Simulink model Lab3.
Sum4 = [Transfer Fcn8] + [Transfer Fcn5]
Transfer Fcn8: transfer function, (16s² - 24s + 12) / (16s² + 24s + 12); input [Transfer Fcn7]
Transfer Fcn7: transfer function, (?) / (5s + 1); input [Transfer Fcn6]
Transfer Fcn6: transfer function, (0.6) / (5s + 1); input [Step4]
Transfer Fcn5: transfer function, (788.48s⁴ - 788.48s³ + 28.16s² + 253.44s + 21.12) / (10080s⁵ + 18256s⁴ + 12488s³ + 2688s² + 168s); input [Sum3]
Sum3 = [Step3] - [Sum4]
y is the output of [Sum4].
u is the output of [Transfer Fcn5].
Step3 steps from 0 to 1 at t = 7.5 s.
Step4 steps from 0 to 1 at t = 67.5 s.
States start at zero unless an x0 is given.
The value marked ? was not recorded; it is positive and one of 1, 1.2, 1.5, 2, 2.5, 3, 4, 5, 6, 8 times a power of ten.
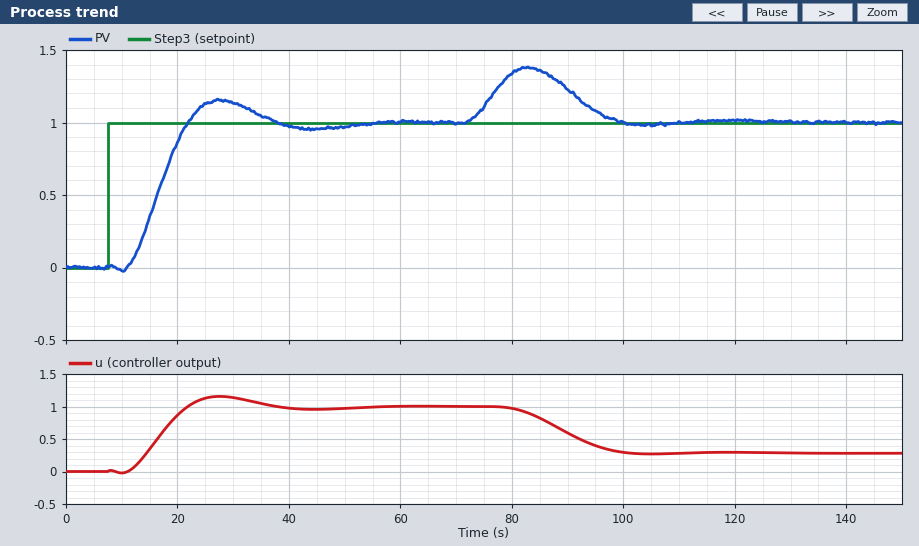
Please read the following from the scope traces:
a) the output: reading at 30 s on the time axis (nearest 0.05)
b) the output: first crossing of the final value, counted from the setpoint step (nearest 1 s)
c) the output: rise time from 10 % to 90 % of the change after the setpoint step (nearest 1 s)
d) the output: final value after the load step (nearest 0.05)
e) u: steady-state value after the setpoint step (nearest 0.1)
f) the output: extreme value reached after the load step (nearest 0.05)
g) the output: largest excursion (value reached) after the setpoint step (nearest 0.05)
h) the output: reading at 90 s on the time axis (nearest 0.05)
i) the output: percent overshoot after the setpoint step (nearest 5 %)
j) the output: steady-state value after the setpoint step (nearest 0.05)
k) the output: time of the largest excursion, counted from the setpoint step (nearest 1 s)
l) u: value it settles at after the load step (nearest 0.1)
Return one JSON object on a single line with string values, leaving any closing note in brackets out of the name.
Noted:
{"the output: reading at 30 s on the time axis": "1.15", "the output: first crossing of the final value, counted from the setpoint step": "14 s", "the output: rise time from 10 % to 90 % of the change after the setpoint step": "8 s", "the output: final value after the load step": "1.00", "u: steady-state value after the setpoint step": "1.0", "the output: extreme value reached after the load step": "1.40", "the output: largest excursion (value reached) after the setpoint step": "1.15", "the output: reading at 90 s on the time axis": "1.25", "the output: percent overshoot after the setpoint step": "15 %", "the output: steady-state value after the setpoint step": "1.00", "the output: time of the largest excursion, counted from the setpoint step": "20 s", "u: value it settles at after the load step": "0.3"}
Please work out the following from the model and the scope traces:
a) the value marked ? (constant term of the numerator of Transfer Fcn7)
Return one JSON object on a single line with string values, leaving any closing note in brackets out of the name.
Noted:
{"the value marked ?": "1.2"}
